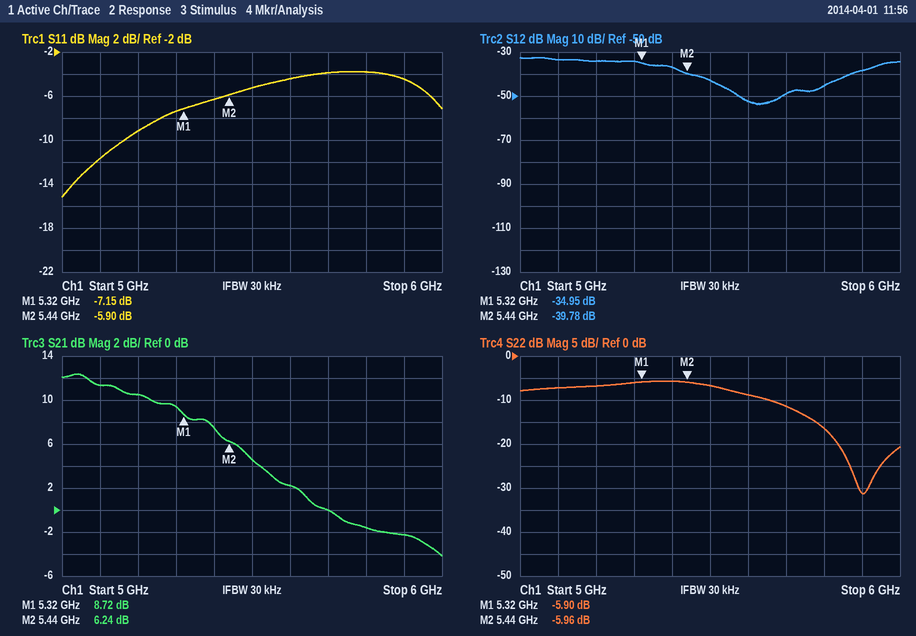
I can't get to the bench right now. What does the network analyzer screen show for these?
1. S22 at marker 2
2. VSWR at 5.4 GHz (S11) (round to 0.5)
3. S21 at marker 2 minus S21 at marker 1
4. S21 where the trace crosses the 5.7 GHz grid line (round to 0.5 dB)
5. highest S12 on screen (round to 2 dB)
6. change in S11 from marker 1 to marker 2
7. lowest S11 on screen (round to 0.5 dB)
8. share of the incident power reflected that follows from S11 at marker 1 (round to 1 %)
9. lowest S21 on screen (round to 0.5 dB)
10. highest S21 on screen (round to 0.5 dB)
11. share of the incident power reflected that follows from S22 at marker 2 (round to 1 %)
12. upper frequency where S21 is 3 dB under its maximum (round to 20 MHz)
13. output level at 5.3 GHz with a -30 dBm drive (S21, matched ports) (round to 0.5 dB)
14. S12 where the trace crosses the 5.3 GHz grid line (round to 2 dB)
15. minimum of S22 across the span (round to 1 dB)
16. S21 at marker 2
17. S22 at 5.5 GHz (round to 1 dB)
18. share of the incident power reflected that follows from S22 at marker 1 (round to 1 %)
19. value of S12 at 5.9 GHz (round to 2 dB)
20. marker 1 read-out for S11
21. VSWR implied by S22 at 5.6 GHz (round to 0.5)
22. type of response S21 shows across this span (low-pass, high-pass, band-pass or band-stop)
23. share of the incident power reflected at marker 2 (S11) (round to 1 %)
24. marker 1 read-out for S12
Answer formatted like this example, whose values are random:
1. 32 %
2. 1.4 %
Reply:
1. -5.96 dB
2. 3.0
3. -2.48 dB
4. 0.0 dB
5. -32 dB
6. 1.25 dB
7. -15.0 dB
8. 19 %
9. -4.0 dB
10. 12.5 dB
11. 25 %
12. 5.30 GHz
13. -20.5 dBm
14. -34 dB
15. -31 dB
16. 6.24 dB
17. -7 dB
18. 26 %
19. -38 dB
20. -7.15 dB
21. 2.0
22. low-pass
23. 26 %
24. -34.95 dB
